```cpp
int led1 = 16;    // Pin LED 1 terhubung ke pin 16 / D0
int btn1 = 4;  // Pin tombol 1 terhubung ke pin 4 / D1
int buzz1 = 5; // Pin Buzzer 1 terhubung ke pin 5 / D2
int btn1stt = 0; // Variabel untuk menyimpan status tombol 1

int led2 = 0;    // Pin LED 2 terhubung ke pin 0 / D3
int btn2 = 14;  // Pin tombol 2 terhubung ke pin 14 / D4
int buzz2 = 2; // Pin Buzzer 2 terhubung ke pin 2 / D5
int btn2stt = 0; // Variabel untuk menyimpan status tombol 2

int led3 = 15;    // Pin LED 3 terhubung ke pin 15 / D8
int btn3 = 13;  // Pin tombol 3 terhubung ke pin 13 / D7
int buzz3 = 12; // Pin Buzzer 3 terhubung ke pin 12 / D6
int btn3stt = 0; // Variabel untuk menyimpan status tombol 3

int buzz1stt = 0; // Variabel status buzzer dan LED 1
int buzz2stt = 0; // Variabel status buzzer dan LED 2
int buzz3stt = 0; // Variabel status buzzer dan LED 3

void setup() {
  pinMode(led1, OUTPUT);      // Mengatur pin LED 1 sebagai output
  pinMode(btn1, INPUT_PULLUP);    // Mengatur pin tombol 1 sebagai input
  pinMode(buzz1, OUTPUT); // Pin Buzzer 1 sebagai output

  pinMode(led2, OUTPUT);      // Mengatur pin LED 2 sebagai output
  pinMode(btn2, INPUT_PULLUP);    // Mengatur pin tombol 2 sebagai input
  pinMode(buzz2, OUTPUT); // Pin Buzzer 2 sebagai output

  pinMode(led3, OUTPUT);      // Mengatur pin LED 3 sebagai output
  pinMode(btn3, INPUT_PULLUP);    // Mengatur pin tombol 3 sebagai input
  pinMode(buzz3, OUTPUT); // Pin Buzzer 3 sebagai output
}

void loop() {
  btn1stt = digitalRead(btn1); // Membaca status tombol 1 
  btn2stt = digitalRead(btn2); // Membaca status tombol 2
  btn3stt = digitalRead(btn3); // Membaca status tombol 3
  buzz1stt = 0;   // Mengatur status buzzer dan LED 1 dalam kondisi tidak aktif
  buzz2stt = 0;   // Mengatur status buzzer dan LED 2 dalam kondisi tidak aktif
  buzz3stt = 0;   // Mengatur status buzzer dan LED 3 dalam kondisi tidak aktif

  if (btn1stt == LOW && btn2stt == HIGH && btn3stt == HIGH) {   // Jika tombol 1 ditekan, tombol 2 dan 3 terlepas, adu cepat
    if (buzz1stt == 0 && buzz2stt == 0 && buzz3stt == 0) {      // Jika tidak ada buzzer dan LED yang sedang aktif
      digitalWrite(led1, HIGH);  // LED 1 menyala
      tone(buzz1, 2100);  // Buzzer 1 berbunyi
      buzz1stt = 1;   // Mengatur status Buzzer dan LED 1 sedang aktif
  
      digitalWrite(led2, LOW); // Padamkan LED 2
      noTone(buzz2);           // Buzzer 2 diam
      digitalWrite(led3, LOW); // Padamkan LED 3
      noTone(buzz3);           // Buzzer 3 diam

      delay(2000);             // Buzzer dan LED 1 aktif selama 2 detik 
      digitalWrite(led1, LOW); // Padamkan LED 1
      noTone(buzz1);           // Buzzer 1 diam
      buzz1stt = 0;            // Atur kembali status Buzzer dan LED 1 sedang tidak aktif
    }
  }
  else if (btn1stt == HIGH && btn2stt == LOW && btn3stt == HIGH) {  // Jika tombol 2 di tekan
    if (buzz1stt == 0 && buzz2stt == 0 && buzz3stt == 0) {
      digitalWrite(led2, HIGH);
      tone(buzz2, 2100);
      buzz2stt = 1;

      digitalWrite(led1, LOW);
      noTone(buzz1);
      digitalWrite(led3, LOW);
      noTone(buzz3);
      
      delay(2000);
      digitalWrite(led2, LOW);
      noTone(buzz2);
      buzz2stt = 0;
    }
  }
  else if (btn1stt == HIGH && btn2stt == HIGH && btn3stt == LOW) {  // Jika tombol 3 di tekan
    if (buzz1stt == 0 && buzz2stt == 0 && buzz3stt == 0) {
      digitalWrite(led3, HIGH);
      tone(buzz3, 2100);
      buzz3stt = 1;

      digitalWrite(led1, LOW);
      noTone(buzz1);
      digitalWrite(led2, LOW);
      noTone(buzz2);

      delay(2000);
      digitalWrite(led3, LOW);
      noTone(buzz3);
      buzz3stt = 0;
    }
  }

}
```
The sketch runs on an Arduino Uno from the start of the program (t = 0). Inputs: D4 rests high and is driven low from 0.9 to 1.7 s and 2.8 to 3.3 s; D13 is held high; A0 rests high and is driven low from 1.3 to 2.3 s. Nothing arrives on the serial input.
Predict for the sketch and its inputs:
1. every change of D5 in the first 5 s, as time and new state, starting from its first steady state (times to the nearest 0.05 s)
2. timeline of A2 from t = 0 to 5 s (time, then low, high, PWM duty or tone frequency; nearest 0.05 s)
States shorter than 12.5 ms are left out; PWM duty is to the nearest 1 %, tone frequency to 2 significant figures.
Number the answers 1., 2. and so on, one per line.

1. 0 s low; 0.9 s tone 2100 Hz; 4.9 s low
2. 0 s low; 0.9 s high; 4.9 s low
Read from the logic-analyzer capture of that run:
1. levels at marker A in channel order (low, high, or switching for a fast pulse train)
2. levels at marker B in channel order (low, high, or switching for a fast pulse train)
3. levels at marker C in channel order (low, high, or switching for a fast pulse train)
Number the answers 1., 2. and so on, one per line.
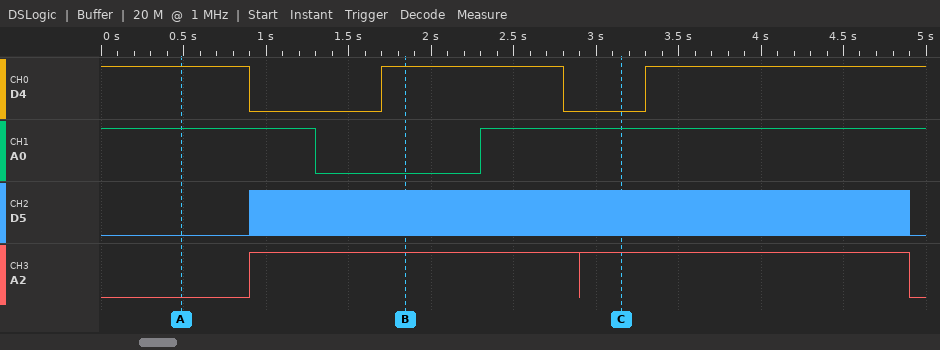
1. D4 high, A0 high, D5 low, A2 low
2. D4 high, A0 low, D5 switching, A2 high
3. D4 low, A0 high, D5 switching, A2 high
